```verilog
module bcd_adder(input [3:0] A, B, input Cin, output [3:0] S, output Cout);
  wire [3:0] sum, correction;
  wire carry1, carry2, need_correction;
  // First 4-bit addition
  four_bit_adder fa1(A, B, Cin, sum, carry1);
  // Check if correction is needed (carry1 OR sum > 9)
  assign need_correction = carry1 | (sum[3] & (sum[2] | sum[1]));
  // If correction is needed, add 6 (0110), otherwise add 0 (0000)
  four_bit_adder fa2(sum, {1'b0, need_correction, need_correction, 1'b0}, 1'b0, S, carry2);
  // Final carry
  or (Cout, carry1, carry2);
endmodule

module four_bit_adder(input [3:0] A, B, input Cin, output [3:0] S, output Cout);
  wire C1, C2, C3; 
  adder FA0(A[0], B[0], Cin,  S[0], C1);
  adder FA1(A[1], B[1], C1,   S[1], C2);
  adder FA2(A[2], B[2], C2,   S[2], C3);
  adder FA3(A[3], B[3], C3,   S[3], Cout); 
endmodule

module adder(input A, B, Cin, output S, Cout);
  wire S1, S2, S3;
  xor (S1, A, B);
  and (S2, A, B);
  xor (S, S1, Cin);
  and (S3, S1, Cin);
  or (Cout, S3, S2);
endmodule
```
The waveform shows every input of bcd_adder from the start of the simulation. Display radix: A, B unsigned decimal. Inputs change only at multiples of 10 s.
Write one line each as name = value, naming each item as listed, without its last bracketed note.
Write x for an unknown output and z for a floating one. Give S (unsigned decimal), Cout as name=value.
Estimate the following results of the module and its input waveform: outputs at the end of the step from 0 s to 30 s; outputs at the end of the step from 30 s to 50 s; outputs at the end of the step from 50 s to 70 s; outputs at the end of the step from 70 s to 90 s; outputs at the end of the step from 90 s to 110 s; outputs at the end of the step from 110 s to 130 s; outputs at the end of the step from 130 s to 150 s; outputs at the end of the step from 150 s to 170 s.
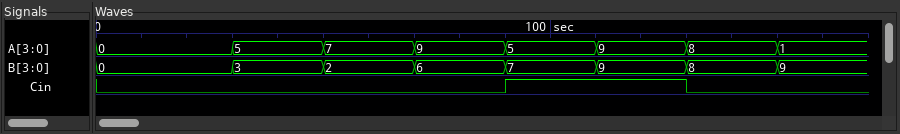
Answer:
outputs at the end of the step from 0 s to 30 s = S=0, Cout=0
outputs at the end of the step from 30 s to 50 s = S=8, Cout=0
outputs at the end of the step from 50 s to 70 s = S=9, Cout=0
outputs at the end of the step from 70 s to 90 s = S=5, Cout=1
outputs at the end of the step from 90 s to 110 s = S=3, Cout=1
outputs at the end of the step from 110 s to 130 s = S=9, Cout=1
outputs at the end of the step from 130 s to 150 s = S=6, Cout=1
outputs at the end of the step from 150 s to 170 s = S=0, Cout=1
